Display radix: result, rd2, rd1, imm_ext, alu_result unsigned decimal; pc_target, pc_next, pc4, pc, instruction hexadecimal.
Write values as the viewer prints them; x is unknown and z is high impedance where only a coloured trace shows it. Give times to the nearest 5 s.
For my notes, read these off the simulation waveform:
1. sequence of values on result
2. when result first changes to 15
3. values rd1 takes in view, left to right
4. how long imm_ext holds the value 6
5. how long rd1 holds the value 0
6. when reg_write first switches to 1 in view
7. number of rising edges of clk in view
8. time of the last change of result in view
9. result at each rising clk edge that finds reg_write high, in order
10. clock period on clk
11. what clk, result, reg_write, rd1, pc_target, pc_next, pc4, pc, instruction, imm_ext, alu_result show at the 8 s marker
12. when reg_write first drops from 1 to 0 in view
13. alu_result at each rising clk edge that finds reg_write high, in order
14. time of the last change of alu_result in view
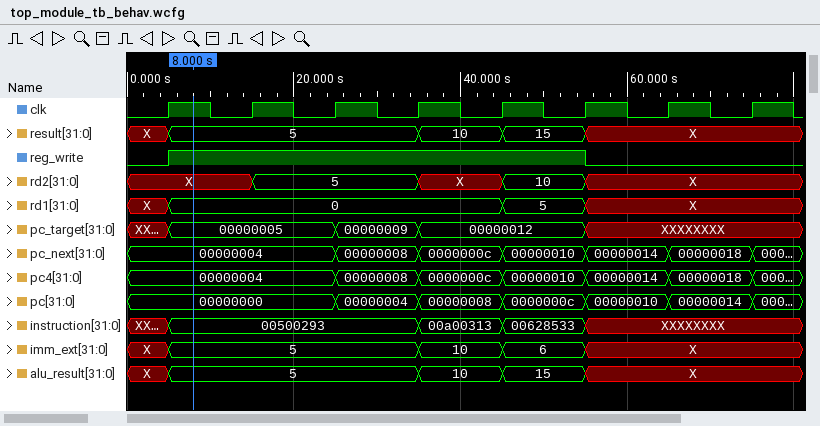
X, 5, 10, 15, X
45 s
X, 0, 5, X
10 s
40 s
5 s
8
55 s
5, 5, 5, 10, 15
10 s
clk=1, result=5, reg_write=1, rd1=0, pc_target=00000005, pc_next=00000004, pc4=00000004, pc=00000000, instruction=00500293, imm_ext=5, alu_result=5
55 s
5, 5, 5, 10, 15
55 s
